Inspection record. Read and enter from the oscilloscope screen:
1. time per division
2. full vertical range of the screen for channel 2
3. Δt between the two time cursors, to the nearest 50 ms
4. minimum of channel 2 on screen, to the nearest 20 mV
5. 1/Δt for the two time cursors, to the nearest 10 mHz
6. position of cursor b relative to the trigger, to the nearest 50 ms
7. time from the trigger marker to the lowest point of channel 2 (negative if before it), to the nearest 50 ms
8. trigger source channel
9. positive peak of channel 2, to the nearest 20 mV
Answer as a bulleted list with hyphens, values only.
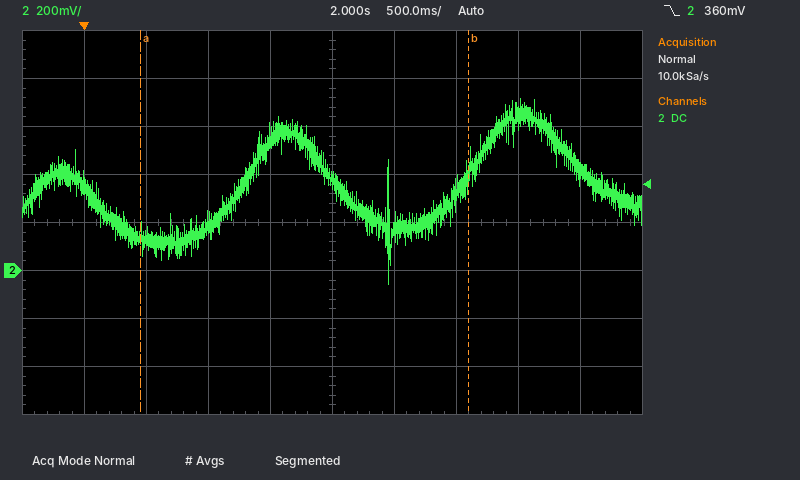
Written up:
- 500 ms
- 1.6 V
- 2.65 s
- -60 mV
- 380 mHz
- +3.10 s
- +2.45 s
- channel 2
- 720 mV
